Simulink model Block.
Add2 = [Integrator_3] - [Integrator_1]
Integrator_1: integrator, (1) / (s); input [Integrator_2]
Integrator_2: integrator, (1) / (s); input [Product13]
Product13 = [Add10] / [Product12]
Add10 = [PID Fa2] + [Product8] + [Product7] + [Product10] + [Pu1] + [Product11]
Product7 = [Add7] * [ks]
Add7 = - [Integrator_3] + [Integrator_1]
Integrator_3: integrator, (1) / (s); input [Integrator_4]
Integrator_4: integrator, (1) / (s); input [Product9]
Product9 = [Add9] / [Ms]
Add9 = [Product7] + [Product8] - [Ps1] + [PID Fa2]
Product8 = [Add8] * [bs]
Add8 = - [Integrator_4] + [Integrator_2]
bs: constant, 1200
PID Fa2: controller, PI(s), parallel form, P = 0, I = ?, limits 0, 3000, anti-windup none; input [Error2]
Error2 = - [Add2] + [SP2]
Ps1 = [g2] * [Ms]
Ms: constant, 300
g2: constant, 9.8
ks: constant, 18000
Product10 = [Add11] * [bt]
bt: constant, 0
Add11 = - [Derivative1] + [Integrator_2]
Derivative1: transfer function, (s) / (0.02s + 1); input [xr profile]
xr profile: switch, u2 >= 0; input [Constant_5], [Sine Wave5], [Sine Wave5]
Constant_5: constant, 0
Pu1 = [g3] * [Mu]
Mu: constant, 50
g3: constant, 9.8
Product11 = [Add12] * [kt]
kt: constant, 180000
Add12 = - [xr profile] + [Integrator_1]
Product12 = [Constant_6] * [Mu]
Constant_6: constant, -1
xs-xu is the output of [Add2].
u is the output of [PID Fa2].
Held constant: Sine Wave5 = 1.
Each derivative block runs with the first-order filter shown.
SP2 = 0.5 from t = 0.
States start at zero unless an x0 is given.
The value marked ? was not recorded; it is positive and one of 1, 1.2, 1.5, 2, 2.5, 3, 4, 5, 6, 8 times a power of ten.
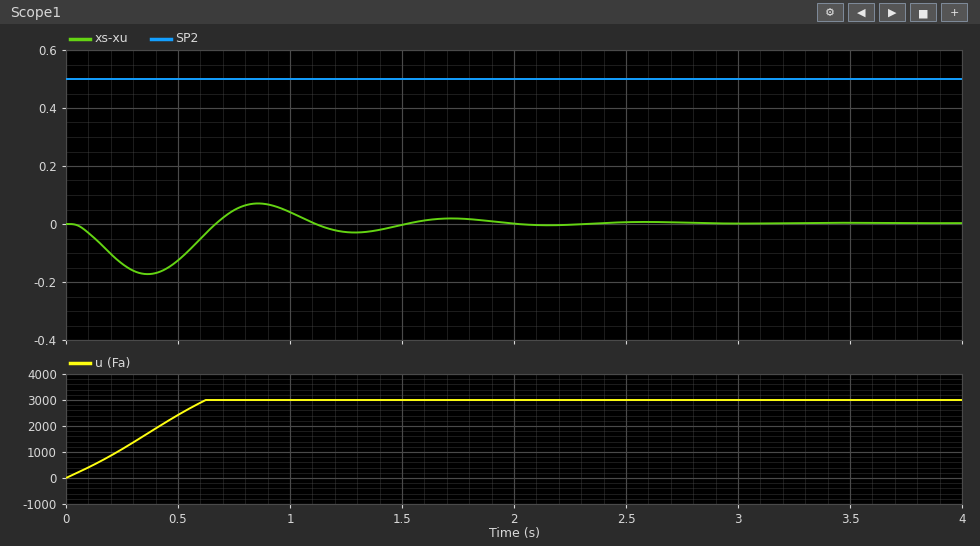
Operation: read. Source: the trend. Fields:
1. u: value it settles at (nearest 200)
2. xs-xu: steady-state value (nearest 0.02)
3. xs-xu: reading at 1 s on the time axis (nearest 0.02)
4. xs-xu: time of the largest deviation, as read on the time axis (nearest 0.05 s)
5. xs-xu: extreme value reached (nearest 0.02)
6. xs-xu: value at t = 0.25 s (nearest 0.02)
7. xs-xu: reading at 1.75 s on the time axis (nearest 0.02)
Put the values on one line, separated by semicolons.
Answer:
3000; 0.00; 0.04; 0.35 s; -0.18; -0.14; 0.02
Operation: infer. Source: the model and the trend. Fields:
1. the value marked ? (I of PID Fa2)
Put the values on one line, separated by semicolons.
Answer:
8000
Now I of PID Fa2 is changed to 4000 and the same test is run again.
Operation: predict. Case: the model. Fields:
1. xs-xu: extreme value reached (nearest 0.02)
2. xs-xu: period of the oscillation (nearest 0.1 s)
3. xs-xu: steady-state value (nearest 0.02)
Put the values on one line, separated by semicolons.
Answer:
-0.20; 0.8 s; 0.00
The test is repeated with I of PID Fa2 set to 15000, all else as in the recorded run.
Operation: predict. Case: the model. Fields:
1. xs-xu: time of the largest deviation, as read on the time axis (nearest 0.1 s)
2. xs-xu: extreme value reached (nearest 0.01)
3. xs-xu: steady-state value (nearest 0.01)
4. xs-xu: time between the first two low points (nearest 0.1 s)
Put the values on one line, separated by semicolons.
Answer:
0.3 s; -0.13; 0.00; 0.9 s
